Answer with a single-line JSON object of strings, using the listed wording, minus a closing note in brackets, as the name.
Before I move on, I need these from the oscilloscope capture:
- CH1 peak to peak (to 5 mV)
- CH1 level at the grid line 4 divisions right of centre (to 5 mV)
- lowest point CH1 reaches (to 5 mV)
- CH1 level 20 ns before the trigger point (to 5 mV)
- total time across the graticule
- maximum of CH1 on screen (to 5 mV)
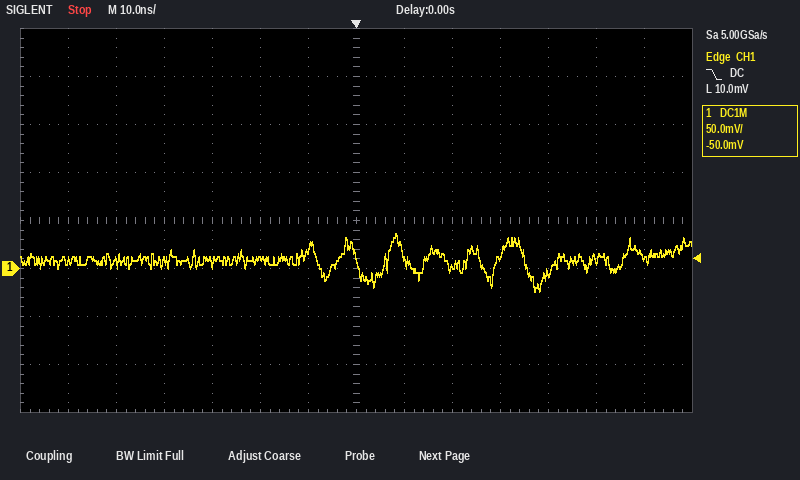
{"CH1 peak to peak": "60 mV", "CH1 level at the grid line 4 divisions right of centre": "-5 mV", "lowest point CH1 reaches": "-25 mV", "CH1 level 20 ns before the trigger point": "10 mV", "total time across the graticule": "140 ns", "maximum of CH1 on screen": "35 mV"}
